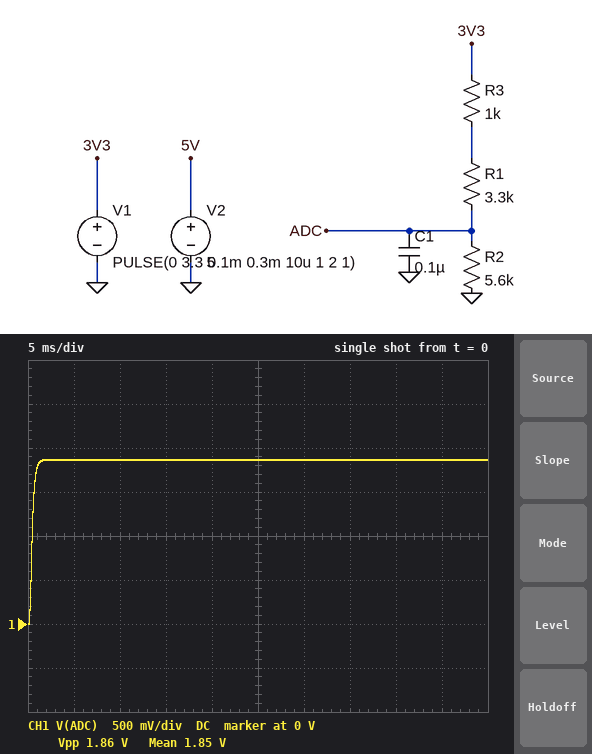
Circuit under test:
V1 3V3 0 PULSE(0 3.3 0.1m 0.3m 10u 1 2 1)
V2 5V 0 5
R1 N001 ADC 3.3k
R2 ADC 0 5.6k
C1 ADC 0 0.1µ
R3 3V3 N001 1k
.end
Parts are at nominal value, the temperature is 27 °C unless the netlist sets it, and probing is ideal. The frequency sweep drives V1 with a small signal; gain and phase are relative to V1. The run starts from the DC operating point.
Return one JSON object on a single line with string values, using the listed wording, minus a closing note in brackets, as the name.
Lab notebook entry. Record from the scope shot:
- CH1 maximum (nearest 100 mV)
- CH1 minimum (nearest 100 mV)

{"CH1 maximum": "1.9 V", "CH1 minimum": "0 V"}
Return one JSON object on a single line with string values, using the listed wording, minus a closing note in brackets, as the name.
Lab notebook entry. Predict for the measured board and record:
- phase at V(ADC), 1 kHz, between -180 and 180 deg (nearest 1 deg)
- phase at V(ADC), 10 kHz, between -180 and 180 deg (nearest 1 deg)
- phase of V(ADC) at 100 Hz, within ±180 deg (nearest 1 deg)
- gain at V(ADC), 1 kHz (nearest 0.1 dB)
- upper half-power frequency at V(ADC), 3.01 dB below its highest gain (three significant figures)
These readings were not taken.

{"phase at V(ADC), 1 kHz, between -180 and 180 deg": "-57 deg", "phase at V(ADC), 10 kHz, between -180 and 180 deg": "-86 deg", "phase of V(ADC) at 100 Hz, within ±180 deg": "-9 deg", "gain at V(ADC), 1 kHz": "-10.2 dB", "upper half-power frequency at V(ADC), 3.01 dB below its highest gain": "654 Hz"}
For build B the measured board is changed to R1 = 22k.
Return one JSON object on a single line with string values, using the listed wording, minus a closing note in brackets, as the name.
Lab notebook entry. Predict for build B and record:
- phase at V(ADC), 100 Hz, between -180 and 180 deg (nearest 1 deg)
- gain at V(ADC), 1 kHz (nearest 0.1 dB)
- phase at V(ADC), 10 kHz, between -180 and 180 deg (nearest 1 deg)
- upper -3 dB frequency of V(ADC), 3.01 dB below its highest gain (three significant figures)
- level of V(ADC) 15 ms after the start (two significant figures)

{"phase at V(ADC), 100 Hz, between -180 and 180 deg": "-16 deg", "gain at V(ADC), 1 kHz": "-23.7 dB", "phase at V(ADC), 10 kHz, between -180 and 180 deg": "-88 deg", "upper -3 dB frequency of V(ADC), 3.01 dB below its highest gain": "353 Hz", "level of V(ADC) 15 ms after the start": "650 mV"}
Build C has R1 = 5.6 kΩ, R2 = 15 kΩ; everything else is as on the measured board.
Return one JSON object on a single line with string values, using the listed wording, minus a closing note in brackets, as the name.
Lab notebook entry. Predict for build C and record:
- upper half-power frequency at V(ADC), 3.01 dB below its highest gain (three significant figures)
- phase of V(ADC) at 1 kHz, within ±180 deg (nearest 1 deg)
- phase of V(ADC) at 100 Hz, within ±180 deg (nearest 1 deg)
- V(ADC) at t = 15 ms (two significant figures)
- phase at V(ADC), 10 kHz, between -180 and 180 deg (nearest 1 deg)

{"upper half-power frequency at V(ADC), 3.01 dB below its highest gain": "347 Hz", "phase of V(ADC) at 1 kHz, within ±180 deg": "-71 deg", "phase of V(ADC) at 100 Hz, within ±180 deg": "-16 deg", "V(ADC) at t = 15 ms": "2.3 V", "phase at V(ADC), 10 kHz, between -180 and 180 deg": "-88 deg"}
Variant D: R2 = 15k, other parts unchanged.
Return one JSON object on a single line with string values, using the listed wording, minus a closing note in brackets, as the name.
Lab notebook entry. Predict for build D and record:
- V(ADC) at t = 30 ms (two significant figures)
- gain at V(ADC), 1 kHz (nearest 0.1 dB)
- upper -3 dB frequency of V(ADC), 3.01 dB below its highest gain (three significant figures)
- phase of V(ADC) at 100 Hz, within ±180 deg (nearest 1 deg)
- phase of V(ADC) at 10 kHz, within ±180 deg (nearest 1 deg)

{"V(ADC) at t = 30 ms": "2.6 V", "gain at V(ADC), 1 kHz": "-9.5 dB", "upper -3 dB frequency of V(ADC), 3.01 dB below its highest gain": "476 Hz", "phase of V(ADC) at 100 Hz, within ±180 deg": "-12 deg", "phase of V(ADC) at 10 kHz, within ±180 deg": "-87 deg"}
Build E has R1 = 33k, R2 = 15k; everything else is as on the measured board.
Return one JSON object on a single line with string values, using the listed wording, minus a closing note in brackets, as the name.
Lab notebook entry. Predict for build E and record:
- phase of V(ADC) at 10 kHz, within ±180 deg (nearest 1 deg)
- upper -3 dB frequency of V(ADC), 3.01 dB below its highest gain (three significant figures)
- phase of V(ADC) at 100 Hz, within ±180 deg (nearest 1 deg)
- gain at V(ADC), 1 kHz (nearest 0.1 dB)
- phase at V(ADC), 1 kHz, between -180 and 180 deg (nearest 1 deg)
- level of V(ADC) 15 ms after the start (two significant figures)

{"phase of V(ADC) at 10 kHz, within ±180 deg": "-89 deg", "upper -3 dB frequency of V(ADC), 3.01 dB below its highest gain": "153 Hz", "phase of V(ADC) at 100 Hz, within ±180 deg": "-33 deg", "gain at V(ADC), 1 kHz": "-26.7 dB", "phase at V(ADC), 1 kHz, between -180 and 180 deg": "-81 deg", "level of V(ADC) 15 ms after the start": "1.0 V"}
